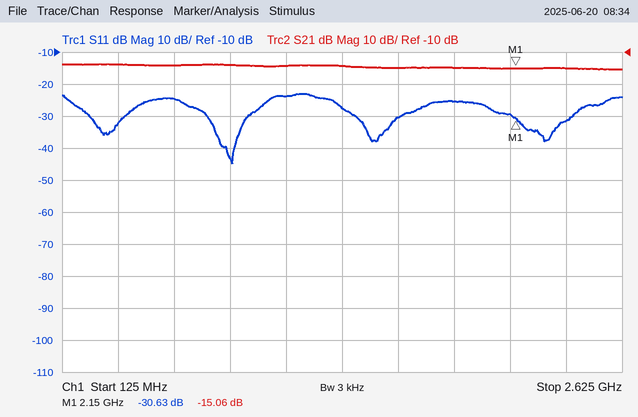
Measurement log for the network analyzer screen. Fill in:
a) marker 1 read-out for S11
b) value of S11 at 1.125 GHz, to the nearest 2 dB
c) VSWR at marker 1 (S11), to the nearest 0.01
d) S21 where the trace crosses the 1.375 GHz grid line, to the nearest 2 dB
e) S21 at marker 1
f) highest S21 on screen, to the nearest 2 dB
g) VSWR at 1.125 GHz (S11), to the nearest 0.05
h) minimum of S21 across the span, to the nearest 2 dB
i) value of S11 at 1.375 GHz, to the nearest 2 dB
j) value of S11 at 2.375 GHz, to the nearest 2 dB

-30.63 dB
-24 dB
1.06
-14 dB
-15.06 dB
-14 dB
1.15
-16 dB
-28 dB
-32 dB
